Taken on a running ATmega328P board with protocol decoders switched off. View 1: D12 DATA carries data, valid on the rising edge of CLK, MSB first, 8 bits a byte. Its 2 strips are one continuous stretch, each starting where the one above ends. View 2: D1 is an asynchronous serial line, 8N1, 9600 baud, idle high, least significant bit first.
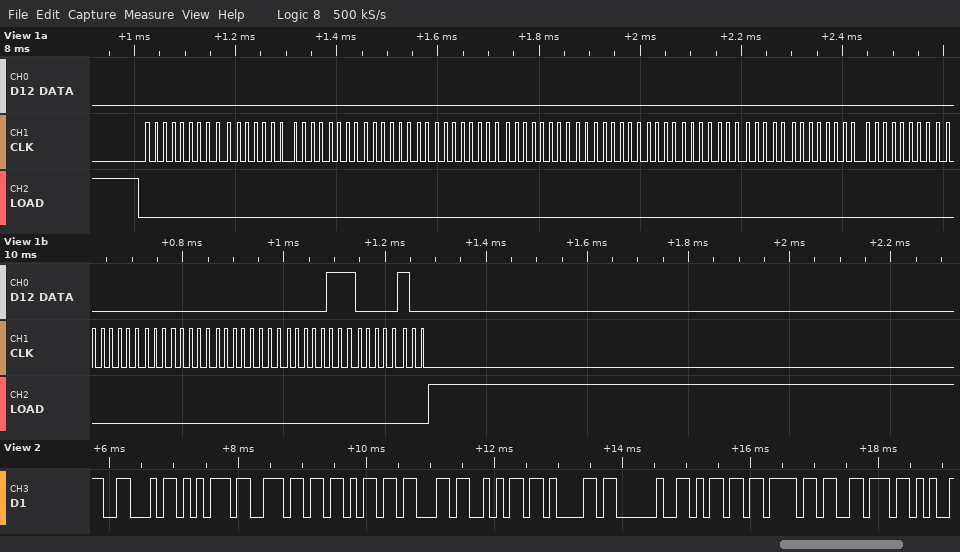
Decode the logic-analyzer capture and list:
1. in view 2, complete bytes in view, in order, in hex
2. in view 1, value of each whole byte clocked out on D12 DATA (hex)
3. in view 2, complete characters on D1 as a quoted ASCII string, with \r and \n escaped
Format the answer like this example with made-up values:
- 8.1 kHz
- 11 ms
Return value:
- 46 75 6E 6B 63 6A 61 20 6D 6F 76
- 0x00 0x00 0x00 0x00 0x00 0x00 0x00 0x00 0x00 0x00 0x00 0x00 0x00 0x00 0x07 0x04
- "Funkcja mov"
